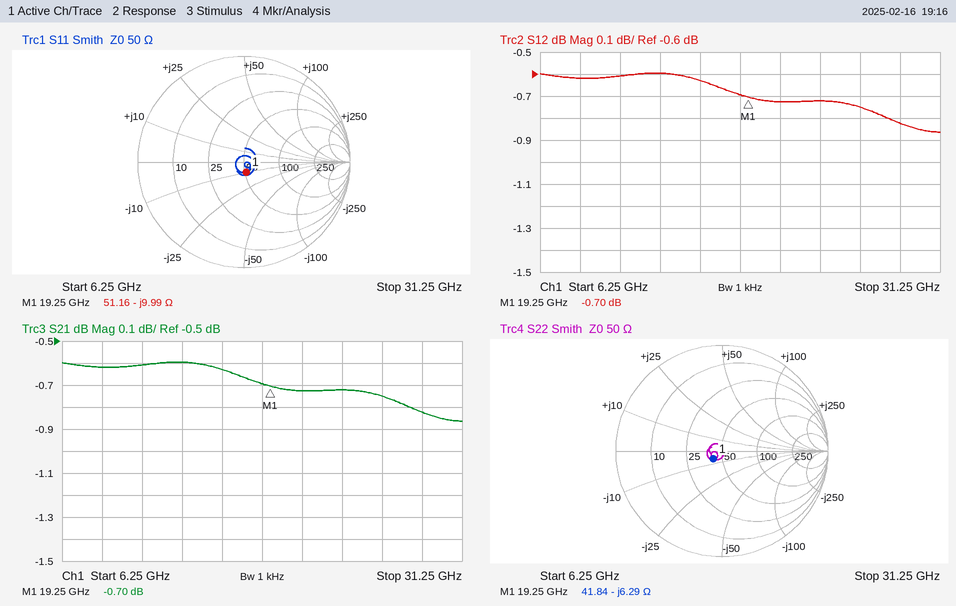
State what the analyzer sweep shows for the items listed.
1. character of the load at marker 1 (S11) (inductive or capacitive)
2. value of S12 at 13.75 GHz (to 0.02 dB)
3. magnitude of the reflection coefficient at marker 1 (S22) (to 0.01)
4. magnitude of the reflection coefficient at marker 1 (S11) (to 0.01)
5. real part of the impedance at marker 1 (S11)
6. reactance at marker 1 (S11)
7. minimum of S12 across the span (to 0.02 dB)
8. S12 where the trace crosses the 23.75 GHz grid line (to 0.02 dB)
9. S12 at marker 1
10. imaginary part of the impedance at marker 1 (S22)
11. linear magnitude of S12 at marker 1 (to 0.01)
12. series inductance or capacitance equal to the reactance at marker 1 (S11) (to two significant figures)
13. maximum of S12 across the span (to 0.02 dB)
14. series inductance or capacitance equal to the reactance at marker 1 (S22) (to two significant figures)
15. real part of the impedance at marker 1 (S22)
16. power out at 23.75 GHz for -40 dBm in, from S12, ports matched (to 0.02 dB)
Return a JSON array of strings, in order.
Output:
["capacitive", "-0.60 dB", "0.11", "0.10", "51.16 Ω", "-9.99 Ω", "-0.86 dB", "-0.72 dB", "-0.70 dB", "-6.29 Ω", "0.92", "830 fF", "-0.60 dB", "1.3 pF", "41.84 Ω", "-40.72 dBm"]
